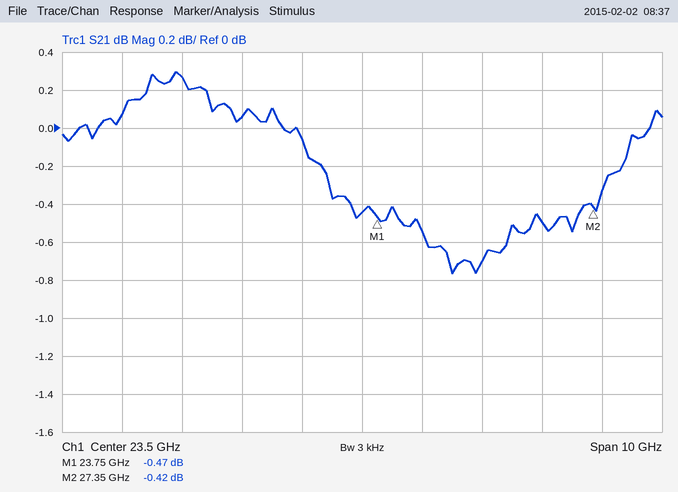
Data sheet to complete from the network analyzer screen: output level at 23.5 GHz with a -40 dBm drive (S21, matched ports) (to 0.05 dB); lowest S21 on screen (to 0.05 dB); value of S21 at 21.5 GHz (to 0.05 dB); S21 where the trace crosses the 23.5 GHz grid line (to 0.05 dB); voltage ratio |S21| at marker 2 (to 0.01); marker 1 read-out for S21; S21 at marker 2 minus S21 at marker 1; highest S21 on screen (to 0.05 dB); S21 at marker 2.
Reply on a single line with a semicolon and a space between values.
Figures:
-40.45 dBm; -0.75 dB; 0.05 dB; -0.45 dB; 0.95; -0.47 dB; 0.05 dB; 0.30 dB; -0.42 dB
